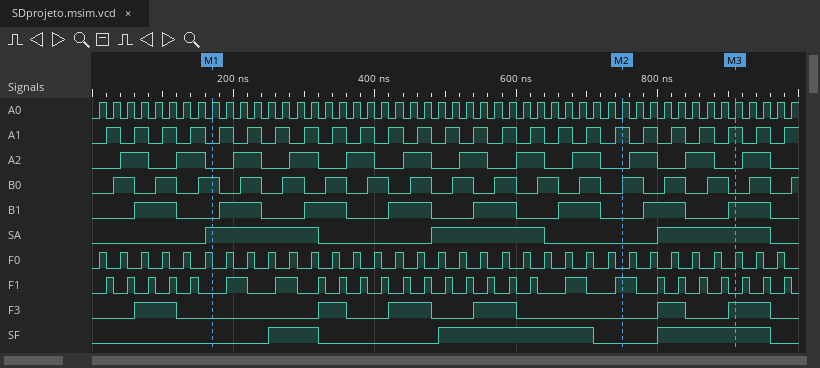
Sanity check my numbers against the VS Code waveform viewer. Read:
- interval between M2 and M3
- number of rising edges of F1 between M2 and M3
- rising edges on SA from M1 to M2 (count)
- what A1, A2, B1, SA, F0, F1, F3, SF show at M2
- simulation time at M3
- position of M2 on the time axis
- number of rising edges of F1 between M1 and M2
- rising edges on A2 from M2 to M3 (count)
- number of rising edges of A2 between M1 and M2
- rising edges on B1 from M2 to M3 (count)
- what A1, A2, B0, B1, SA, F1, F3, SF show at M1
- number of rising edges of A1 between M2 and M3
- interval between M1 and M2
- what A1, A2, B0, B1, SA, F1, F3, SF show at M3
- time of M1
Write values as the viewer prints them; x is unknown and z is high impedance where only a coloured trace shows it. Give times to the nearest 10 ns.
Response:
160 ns
4
1
A1=1, A2=0, B1=0, SA=0, F0=0, F1=1, F3=0, SF=0
910 ns
750 ns
15
2
7
2
A1=0, A2=0, B0=1, B1=0, SA=1, F1=0, F3=0, SF=0
4
580 ns
A1=1, A2=0, B0=0, B1=1, SA=1, F1=0, F3=1, SF=1
170 ns
